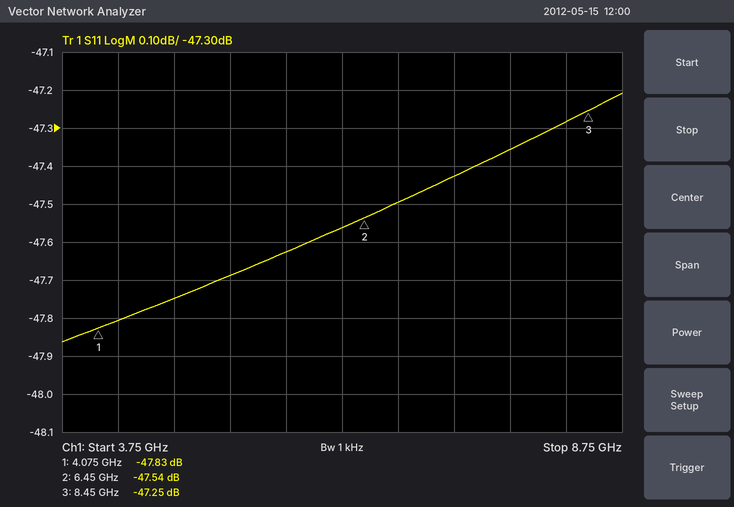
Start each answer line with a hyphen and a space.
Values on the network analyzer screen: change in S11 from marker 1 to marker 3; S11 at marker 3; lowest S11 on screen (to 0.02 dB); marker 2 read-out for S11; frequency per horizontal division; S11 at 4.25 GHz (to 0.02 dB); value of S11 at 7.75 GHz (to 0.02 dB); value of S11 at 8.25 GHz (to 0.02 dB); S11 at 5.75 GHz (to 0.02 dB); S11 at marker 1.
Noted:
- 0.58 dB
- -47.25 dB
- -47.86 dB
- -47.54 dB
- 500 MHz
- -47.80 dB
- -47.36 dB
- -47.28 dB
- -47.62 dB
- -47.83 dB
